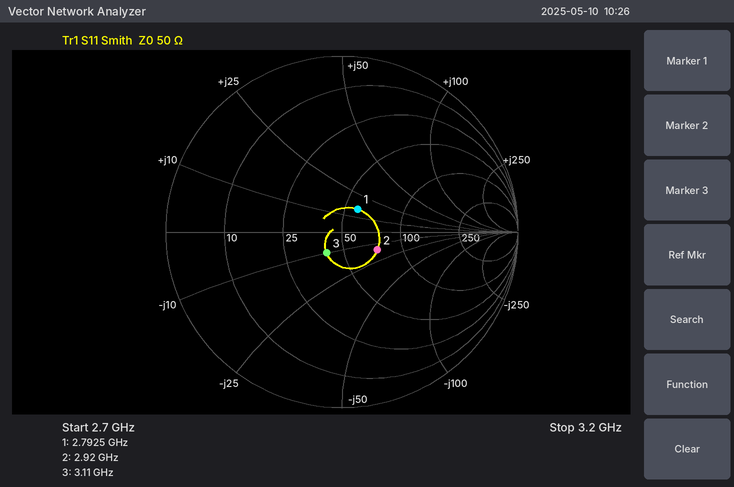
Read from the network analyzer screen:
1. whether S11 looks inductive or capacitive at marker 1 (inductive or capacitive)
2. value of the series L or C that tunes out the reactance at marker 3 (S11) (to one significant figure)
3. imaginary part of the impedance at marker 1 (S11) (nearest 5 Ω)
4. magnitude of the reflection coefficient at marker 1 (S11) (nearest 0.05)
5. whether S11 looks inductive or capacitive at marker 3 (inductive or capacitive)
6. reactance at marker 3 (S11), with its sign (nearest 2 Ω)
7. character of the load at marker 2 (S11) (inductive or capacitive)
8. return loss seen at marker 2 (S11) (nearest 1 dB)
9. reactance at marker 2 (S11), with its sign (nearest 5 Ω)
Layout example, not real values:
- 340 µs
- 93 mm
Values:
- inductive
- 500 pH
- +15 Ω
- 0.15
- capacitive
- -10 Ω
- capacitive
- 13 dB
- -15 Ω
